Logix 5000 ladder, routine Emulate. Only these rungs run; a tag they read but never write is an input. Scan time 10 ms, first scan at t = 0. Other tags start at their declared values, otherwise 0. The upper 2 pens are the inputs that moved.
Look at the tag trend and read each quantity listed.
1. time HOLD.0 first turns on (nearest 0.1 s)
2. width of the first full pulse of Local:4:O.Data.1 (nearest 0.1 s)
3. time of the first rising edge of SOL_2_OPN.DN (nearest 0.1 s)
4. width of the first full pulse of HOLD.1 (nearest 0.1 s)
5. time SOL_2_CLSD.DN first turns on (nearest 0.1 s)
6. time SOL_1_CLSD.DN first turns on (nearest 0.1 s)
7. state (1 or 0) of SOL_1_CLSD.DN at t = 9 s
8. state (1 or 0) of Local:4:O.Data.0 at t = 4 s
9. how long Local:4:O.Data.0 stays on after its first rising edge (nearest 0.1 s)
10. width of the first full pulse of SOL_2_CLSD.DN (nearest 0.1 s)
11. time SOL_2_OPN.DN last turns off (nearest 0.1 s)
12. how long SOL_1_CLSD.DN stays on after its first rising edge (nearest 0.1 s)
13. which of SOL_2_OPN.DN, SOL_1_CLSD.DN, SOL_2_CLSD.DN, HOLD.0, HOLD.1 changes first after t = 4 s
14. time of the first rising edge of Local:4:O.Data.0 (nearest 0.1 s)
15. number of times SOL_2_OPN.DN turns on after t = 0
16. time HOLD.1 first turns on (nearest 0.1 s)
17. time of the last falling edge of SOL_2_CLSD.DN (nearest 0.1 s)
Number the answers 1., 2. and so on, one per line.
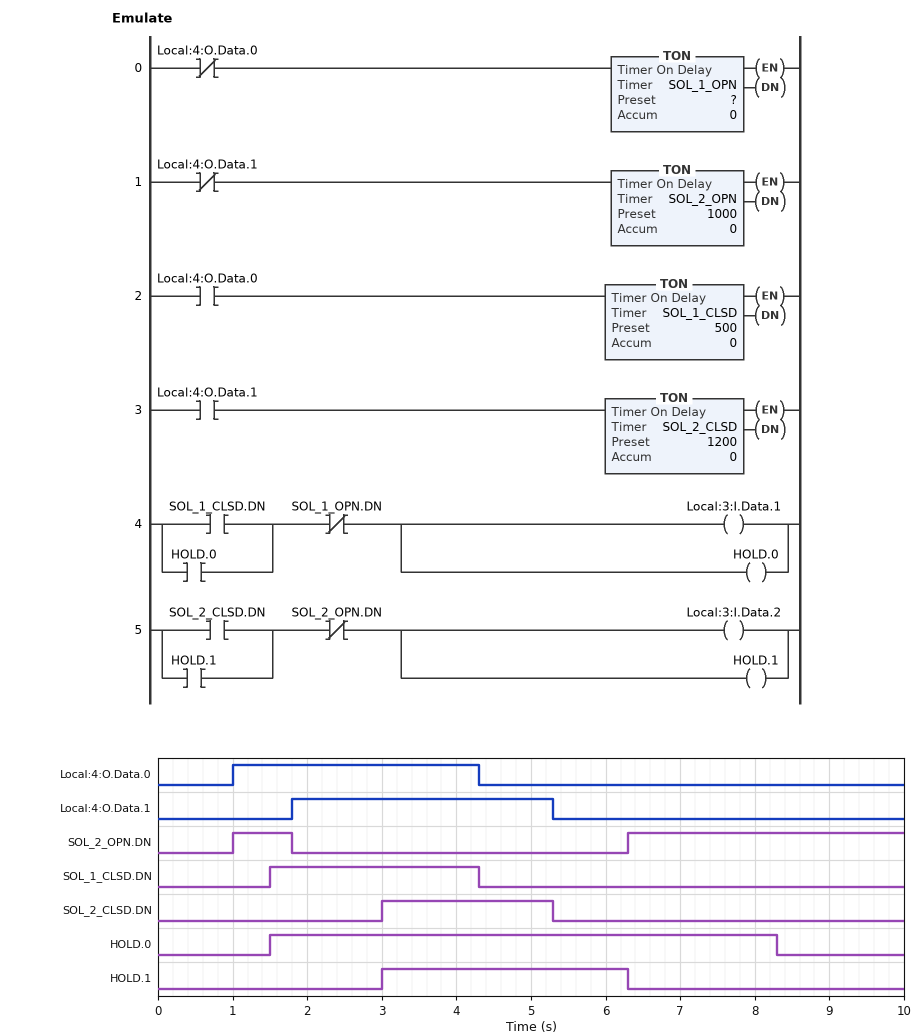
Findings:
1. 1.5 s
2. 3.5 s
3. 1.0 s
4. 3.3 s
5. 3.0 s
6. 1.5 s
7. 0
8. 1
9. 3.3 s
10. 2.3 s
11. 1.8 s
12. 2.8 s
13. SOL_1_CLSD.DN
14. 1.0 s
15. 2
16. 3.0 s
17. 5.3 s
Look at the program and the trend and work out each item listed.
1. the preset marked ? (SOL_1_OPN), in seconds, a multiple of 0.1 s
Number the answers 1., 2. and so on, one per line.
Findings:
1. 4.0 s
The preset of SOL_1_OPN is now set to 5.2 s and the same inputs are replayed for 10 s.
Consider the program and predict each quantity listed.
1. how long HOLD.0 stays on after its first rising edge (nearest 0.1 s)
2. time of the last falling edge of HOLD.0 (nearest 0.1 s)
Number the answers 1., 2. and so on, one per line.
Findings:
1. 8.0 s
2. 9.5 s
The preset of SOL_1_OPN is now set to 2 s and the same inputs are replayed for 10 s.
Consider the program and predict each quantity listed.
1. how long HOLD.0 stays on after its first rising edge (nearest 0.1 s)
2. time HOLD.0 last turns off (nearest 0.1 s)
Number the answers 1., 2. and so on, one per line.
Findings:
1. 4.8 s
2. 6.3 s
